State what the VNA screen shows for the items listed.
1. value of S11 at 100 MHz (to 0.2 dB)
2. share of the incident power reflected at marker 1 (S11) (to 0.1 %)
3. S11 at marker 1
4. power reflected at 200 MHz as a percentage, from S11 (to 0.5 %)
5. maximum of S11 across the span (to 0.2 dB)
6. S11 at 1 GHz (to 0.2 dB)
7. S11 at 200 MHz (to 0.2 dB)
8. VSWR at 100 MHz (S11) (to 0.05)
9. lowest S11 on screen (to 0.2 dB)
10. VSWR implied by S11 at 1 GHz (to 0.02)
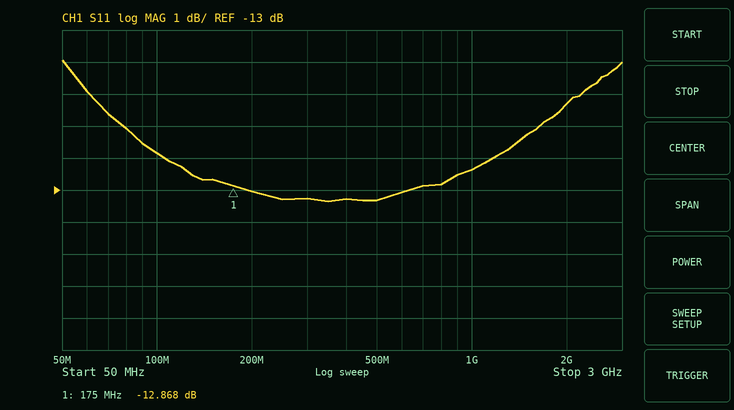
-11.8 dB
5.2 %
-12.868 dB
5.0 %
-9.0 dB
-12.4 dB
-13.0 dB
1.70
-13.4 dB
1.64
